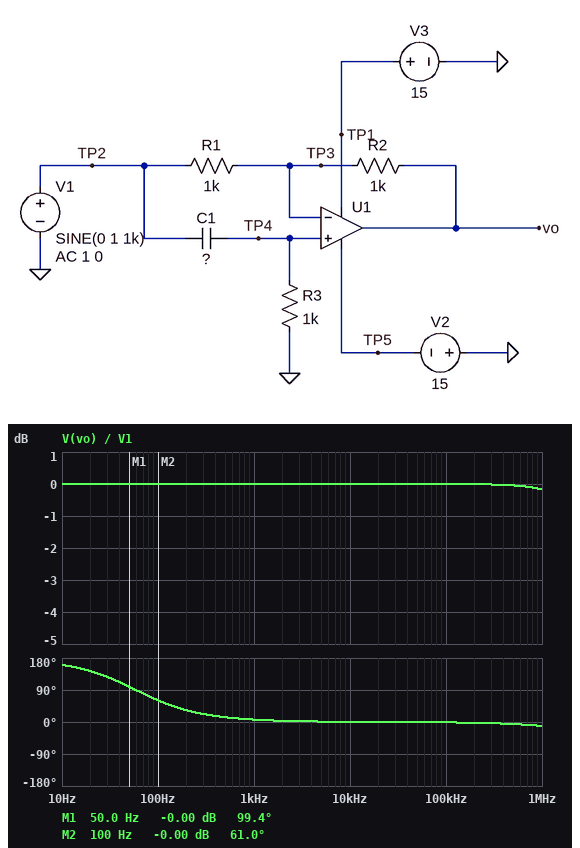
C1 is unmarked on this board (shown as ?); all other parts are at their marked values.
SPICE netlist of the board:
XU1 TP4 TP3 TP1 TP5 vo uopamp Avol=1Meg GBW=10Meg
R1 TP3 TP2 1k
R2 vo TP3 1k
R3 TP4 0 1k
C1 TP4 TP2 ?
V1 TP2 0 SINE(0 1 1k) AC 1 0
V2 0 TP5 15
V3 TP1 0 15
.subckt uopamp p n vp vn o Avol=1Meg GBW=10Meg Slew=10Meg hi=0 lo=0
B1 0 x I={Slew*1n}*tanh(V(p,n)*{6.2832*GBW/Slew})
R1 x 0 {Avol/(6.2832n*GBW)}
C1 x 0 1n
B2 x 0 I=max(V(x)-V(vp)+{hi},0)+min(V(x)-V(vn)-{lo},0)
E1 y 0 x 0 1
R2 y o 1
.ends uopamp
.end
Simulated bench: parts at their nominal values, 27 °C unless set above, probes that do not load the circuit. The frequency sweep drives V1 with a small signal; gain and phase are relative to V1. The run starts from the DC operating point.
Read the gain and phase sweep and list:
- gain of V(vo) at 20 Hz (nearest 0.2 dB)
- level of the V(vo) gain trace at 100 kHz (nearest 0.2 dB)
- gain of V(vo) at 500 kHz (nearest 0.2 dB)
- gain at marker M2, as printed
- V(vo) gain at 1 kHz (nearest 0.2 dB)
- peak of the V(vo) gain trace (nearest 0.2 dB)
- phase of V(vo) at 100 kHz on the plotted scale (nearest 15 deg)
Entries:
0 dB
0 dB
0 dB
-0.00 dB
0 dB
0 dB
0 deg
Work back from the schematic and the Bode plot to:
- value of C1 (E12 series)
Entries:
2.7 µF
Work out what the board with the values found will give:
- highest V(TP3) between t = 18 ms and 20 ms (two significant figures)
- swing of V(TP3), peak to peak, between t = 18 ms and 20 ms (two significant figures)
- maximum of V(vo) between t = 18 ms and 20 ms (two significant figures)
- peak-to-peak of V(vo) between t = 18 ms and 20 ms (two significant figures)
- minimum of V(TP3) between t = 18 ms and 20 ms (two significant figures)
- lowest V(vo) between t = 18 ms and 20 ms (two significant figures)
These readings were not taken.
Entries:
1.0 V
2.0 V
1.0 V
2.0 V
-1.0 V
-1.0 V
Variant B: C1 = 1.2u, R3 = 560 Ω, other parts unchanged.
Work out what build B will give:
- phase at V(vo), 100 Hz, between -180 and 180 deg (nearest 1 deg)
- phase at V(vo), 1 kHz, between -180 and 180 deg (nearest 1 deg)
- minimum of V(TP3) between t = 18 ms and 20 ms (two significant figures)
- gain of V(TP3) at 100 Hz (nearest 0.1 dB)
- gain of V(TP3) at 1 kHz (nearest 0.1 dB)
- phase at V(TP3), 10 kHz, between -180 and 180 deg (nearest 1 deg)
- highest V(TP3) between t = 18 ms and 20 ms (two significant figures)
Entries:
134 deg
27 deg
-970 mV
-8.2 dB
-0.2 dB
1 deg
970 mV
